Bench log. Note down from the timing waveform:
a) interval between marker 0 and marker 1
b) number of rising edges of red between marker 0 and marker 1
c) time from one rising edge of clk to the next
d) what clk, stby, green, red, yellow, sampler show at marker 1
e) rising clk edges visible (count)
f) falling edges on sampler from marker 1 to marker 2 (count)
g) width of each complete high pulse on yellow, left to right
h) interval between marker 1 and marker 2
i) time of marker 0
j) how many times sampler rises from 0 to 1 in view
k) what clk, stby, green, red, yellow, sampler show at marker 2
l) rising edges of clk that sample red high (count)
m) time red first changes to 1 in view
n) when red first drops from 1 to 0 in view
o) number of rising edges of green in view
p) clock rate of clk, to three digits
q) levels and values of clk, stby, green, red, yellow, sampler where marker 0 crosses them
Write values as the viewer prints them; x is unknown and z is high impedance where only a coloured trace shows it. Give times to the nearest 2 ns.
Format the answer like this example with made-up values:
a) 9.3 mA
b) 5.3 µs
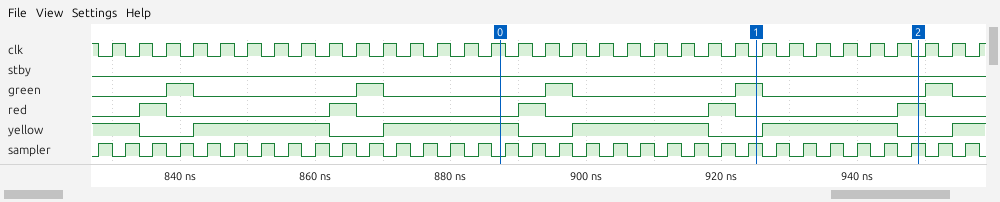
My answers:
a) 38 ns
b) 2
c) 4 ns
d) clk=0, stby=0, green=1, red=0, yellow=0, sampler=1
e) 33
f) 6
g) 20 ns, 20 ns, 20 ns, 20 ns
h) 24 ns
i) 888 ns
j) 33
k) clk=0, stby=0, green=0, red=1, yellow=0, sampler=1
l) 5
m) 834 ns
n) 838 ns
o) 5
p) 250 MHz
q) clk=1, stby=0, green=0, red=0, yellow=1, sampler=0
